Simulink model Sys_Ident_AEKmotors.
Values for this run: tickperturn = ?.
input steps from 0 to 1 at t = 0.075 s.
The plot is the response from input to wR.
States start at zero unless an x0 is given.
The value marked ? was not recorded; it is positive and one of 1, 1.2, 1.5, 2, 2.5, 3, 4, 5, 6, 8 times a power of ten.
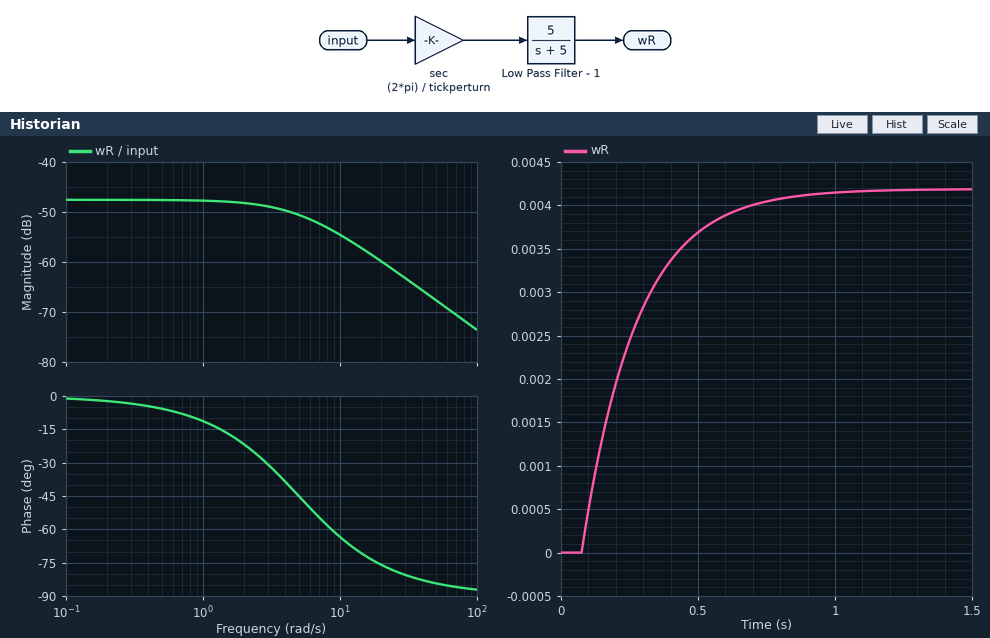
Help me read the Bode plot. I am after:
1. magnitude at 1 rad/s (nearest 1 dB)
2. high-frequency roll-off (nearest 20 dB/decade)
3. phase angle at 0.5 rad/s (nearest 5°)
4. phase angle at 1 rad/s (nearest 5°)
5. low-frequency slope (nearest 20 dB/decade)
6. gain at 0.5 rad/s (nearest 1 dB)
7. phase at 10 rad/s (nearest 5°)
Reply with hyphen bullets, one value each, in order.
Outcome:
- -48 dB
- -20 dB/decade
- -5°
- -10°
- 0 dB/decade
- -48 dB
- -65°
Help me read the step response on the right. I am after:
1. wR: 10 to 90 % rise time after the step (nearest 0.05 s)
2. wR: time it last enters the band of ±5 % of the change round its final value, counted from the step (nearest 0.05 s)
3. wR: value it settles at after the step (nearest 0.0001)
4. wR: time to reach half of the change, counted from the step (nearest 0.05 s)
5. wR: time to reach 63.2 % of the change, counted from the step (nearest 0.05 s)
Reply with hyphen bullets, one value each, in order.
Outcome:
- 0.45 s
- 0.60 s
- 0.0042
- 0.15 s
- 0.20 s
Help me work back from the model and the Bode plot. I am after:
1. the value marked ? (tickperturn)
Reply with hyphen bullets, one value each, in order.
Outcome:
- 1500
